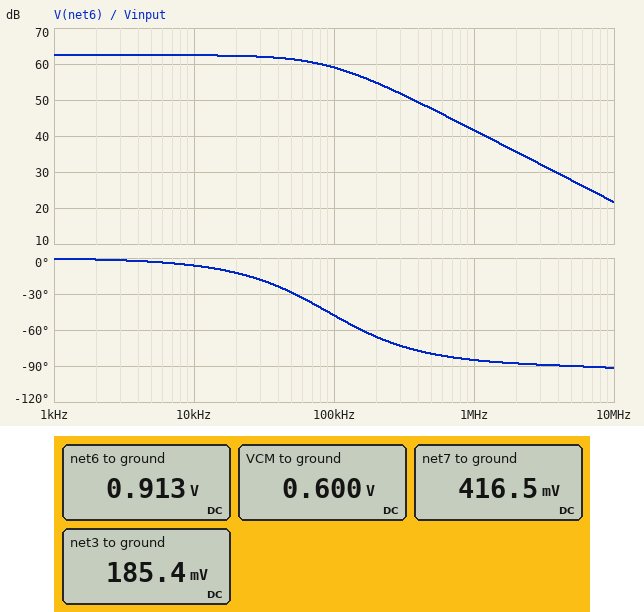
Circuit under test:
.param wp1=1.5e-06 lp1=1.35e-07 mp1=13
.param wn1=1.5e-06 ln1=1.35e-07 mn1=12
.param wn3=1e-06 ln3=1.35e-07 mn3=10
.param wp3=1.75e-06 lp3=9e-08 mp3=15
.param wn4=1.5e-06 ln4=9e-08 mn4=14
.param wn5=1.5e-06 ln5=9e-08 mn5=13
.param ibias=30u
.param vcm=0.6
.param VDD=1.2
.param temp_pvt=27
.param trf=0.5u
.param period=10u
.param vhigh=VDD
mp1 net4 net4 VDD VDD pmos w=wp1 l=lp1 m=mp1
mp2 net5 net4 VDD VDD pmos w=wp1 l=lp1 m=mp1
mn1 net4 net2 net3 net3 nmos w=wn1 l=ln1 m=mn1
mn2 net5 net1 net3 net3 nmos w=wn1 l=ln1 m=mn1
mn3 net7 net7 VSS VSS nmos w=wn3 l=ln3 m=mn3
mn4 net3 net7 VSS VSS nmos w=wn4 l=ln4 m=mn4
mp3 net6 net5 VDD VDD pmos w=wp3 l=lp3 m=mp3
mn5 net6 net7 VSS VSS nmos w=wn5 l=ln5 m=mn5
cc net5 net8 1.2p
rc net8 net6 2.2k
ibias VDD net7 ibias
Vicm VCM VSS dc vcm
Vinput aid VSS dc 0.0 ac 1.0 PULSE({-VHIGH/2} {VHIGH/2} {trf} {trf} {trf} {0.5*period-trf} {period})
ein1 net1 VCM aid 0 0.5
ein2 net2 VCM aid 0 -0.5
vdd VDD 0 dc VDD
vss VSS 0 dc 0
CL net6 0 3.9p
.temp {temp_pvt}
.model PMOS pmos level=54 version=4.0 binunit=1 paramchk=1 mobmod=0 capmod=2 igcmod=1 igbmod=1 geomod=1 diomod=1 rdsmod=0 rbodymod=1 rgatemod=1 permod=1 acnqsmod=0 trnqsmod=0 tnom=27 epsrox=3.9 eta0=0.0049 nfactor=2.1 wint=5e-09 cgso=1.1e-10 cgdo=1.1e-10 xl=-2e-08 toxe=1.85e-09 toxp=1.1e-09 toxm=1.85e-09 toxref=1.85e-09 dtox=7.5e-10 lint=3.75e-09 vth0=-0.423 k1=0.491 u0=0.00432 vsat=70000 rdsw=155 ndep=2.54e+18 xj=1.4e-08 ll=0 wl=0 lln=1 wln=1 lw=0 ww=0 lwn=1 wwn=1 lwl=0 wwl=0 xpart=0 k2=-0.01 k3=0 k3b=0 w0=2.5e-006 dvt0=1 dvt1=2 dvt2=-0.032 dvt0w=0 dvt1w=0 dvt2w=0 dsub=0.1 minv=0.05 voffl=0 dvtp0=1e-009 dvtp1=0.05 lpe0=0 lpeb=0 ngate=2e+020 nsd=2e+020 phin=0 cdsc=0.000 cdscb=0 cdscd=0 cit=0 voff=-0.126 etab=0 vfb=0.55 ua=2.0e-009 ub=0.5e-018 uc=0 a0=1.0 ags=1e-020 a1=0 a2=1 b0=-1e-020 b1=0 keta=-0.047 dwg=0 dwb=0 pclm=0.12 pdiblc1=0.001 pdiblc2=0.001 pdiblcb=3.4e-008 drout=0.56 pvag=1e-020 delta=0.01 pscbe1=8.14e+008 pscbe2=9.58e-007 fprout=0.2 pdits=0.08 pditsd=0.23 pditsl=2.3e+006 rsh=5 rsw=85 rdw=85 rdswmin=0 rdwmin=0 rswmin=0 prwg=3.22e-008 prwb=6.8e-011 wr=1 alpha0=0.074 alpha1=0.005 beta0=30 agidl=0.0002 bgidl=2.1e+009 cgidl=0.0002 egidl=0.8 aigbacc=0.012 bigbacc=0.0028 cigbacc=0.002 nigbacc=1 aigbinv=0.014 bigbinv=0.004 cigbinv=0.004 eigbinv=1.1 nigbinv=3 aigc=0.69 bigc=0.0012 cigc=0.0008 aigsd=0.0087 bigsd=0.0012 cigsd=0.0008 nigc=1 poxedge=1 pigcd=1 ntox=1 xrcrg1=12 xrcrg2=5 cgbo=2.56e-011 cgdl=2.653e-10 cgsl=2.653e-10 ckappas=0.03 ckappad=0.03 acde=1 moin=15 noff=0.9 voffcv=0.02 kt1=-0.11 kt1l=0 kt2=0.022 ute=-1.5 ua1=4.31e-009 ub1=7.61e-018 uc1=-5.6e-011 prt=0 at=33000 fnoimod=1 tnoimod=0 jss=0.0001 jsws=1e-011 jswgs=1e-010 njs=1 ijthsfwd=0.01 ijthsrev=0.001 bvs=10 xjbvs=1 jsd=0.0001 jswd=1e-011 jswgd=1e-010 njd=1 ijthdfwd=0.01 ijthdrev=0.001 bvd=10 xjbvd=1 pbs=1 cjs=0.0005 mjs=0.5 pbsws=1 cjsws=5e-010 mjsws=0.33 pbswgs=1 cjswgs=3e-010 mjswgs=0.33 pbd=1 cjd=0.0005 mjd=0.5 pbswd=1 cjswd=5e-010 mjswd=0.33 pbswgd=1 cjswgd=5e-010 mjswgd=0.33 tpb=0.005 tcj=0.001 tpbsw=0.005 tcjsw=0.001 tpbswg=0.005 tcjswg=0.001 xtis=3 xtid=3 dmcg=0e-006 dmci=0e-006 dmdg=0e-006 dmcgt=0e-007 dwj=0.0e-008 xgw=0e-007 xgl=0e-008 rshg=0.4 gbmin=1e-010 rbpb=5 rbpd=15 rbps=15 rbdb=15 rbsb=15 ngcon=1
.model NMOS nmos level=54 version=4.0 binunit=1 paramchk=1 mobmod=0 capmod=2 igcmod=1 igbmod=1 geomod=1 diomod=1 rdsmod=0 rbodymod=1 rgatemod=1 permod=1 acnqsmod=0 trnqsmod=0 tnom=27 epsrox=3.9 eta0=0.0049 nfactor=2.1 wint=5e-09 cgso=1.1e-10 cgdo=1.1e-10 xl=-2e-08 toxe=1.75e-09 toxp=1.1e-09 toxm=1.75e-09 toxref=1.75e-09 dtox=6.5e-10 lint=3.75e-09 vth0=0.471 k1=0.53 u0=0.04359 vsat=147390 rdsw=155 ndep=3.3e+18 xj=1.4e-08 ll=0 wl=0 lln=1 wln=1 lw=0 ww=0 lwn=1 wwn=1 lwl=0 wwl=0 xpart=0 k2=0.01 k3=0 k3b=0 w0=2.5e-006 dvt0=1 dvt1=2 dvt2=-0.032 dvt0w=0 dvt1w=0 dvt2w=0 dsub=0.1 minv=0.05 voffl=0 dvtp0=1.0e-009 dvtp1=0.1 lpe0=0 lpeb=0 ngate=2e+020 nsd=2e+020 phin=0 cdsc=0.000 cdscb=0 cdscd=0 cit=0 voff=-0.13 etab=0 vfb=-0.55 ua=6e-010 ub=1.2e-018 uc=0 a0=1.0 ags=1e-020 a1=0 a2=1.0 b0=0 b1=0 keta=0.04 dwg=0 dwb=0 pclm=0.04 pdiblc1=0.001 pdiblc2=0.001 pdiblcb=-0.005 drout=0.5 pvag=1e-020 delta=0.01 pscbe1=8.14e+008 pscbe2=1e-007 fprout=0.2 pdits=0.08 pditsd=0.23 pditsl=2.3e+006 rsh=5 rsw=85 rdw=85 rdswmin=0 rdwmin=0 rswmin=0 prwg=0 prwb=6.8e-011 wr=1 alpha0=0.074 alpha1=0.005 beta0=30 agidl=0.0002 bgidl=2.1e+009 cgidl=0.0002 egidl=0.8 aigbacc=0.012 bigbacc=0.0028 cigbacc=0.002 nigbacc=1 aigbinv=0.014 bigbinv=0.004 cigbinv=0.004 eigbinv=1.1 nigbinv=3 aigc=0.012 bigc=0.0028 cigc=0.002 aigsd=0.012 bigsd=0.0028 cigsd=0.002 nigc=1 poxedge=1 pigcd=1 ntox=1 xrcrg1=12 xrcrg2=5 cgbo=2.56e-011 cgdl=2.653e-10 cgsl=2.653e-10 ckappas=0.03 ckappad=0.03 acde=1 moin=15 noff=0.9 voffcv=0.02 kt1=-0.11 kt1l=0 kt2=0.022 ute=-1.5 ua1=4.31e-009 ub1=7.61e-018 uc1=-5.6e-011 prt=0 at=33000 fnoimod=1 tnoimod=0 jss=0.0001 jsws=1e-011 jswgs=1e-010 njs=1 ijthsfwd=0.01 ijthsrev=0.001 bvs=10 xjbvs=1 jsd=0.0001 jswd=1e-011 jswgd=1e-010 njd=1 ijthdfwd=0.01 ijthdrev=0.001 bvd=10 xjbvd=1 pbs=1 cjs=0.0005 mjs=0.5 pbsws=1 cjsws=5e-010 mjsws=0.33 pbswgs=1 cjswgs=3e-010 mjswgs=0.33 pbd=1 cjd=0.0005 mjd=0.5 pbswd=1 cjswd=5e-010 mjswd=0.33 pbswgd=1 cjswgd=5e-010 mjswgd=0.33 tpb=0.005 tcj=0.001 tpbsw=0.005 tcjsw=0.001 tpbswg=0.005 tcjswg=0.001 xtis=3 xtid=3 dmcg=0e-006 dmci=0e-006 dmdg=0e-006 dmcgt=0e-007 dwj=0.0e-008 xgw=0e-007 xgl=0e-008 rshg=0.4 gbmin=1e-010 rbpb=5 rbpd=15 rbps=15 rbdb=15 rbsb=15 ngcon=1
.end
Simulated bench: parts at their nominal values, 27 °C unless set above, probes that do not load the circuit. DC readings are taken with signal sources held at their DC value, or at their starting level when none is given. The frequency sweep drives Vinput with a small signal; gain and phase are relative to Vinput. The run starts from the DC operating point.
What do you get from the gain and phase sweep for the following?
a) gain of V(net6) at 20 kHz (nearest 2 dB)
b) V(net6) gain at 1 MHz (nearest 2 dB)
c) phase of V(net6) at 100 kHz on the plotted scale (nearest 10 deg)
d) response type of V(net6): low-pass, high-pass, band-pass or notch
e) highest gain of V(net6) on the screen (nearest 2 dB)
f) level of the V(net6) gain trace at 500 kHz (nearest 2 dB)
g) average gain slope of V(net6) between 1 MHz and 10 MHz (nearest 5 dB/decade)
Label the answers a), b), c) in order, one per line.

a) 62 dB
b) 42 dB
c) -50 deg
d) low-pass
e) 62 dB
f) 48 dB
g) -20 dB/decade
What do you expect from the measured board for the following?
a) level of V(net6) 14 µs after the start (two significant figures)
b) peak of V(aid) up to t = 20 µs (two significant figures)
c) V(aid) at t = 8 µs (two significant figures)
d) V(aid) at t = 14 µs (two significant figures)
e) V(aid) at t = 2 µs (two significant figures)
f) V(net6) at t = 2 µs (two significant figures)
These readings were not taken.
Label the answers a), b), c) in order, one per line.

a) 1.2 V
b) 600 mV
c) -600 mV
d) 600 mV
e) 600 mV
f) 1.2 V
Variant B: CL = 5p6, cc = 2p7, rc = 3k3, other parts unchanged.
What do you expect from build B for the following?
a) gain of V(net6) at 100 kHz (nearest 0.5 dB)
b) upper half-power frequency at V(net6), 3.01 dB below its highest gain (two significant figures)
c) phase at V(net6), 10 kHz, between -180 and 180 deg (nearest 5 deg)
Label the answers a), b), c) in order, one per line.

a) 54.0 dB
b) 41 kHz
c) -15 deg
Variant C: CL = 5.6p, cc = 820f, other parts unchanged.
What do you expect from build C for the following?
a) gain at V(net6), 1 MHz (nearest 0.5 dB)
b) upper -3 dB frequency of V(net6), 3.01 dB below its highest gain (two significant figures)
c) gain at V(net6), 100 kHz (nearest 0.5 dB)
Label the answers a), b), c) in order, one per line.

a) 44.5 dB
b) 130 kHz
c) 60.5 dB
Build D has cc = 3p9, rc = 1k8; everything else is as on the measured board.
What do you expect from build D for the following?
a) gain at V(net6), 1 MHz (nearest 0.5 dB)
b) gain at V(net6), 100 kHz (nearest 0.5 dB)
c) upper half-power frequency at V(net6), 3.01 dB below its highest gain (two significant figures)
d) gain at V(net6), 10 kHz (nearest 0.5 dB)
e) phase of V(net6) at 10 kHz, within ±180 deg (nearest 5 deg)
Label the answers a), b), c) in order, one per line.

a) 31.5 dB
b) 51.5 dB
c) 29 kHz
d) 62.0 dB
e) -20 deg
